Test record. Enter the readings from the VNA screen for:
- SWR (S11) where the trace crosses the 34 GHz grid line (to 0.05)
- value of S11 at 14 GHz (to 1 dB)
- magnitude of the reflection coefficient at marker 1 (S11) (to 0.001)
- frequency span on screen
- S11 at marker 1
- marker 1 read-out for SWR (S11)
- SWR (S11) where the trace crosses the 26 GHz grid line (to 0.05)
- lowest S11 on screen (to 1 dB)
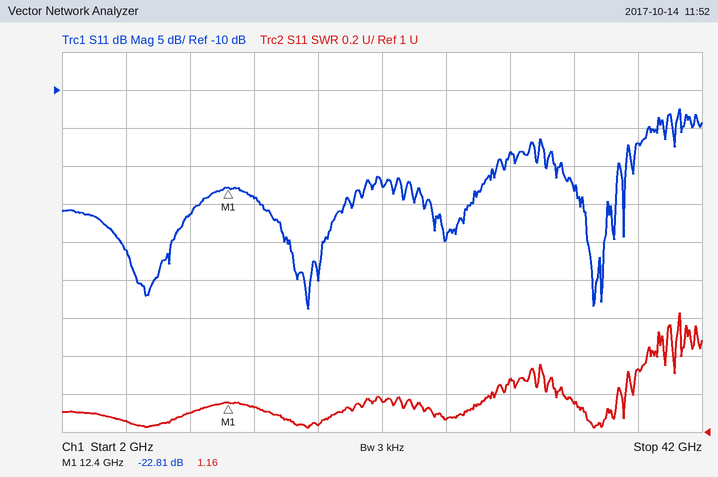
1.15
-24 dB
0.072
40 GHz
-22.81 dB
1.16
1.05
-39 dB
